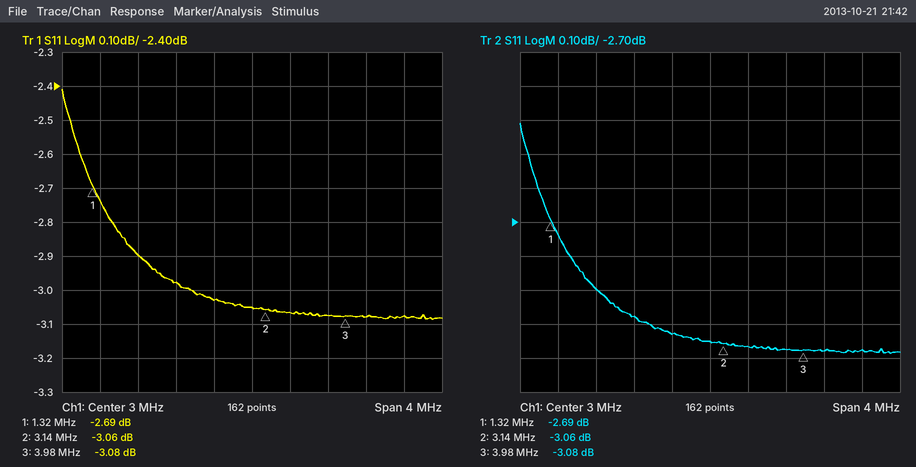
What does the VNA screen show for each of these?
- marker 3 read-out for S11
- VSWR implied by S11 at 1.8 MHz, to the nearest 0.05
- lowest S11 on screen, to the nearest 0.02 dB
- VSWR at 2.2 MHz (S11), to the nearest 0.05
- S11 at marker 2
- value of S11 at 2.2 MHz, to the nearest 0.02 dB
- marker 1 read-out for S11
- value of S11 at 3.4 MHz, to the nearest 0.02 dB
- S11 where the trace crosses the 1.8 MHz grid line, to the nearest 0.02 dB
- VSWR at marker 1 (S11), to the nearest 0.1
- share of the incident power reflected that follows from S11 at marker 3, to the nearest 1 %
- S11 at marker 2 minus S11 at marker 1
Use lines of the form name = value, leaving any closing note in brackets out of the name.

marker 3 read-out for S11 = -3.08 dB
VSWR implied by S11 at 1.8 MHz, to the nearest 0.05 = 6.05
lowest S11 on screen, to the nearest 0.02 dB = -3.08 dB
VSWR at 2.2 MHz (S11), to the nearest 0.05 = 5.90
S11 at marker 2 = -3.06 dB
value of S11 at 2.2 MHz, to the nearest 0.02 dB = -2.98 dB
marker 1 read-out for S11 = -2.69 dB
value of S11 at 3.4 MHz, to the nearest 0.02 dB = -3.06 dB
S11 where the trace crosses the 1.8 MHz grid line, to the nearest 0.02 dB = -2.90 dB
VSWR at marker 1 (S11), to the nearest 0.1 = 6.5
share of the incident power reflected that follows from S11 at marker 3, to the nearest 1 % = 49 %
S11 at marker 2 minus S11 at marker 1 = -0.37 dB
